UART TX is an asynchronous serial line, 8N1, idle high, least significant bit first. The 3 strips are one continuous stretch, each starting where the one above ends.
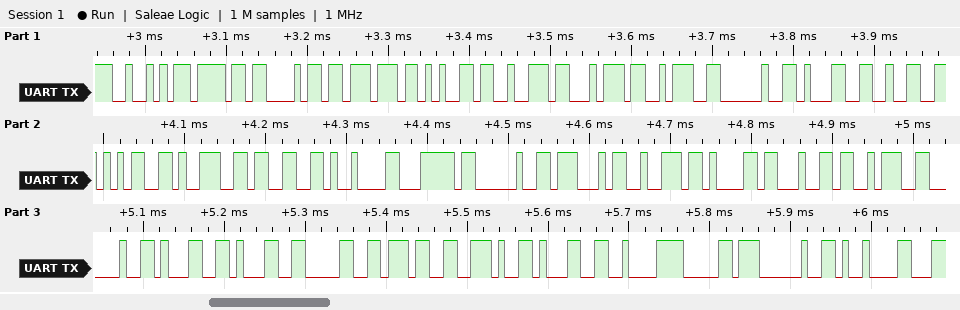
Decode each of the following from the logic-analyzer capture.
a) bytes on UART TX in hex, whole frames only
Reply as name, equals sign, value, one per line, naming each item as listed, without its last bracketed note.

bytes on UART TX in hex, whole frames only = 52 6F 68 77 65 72 74 3A 20 31 32 35 39 33 09 7C 20 47 72 61 64 3A 20 31 31 30 37 2E 31 C2 B0 20 09
